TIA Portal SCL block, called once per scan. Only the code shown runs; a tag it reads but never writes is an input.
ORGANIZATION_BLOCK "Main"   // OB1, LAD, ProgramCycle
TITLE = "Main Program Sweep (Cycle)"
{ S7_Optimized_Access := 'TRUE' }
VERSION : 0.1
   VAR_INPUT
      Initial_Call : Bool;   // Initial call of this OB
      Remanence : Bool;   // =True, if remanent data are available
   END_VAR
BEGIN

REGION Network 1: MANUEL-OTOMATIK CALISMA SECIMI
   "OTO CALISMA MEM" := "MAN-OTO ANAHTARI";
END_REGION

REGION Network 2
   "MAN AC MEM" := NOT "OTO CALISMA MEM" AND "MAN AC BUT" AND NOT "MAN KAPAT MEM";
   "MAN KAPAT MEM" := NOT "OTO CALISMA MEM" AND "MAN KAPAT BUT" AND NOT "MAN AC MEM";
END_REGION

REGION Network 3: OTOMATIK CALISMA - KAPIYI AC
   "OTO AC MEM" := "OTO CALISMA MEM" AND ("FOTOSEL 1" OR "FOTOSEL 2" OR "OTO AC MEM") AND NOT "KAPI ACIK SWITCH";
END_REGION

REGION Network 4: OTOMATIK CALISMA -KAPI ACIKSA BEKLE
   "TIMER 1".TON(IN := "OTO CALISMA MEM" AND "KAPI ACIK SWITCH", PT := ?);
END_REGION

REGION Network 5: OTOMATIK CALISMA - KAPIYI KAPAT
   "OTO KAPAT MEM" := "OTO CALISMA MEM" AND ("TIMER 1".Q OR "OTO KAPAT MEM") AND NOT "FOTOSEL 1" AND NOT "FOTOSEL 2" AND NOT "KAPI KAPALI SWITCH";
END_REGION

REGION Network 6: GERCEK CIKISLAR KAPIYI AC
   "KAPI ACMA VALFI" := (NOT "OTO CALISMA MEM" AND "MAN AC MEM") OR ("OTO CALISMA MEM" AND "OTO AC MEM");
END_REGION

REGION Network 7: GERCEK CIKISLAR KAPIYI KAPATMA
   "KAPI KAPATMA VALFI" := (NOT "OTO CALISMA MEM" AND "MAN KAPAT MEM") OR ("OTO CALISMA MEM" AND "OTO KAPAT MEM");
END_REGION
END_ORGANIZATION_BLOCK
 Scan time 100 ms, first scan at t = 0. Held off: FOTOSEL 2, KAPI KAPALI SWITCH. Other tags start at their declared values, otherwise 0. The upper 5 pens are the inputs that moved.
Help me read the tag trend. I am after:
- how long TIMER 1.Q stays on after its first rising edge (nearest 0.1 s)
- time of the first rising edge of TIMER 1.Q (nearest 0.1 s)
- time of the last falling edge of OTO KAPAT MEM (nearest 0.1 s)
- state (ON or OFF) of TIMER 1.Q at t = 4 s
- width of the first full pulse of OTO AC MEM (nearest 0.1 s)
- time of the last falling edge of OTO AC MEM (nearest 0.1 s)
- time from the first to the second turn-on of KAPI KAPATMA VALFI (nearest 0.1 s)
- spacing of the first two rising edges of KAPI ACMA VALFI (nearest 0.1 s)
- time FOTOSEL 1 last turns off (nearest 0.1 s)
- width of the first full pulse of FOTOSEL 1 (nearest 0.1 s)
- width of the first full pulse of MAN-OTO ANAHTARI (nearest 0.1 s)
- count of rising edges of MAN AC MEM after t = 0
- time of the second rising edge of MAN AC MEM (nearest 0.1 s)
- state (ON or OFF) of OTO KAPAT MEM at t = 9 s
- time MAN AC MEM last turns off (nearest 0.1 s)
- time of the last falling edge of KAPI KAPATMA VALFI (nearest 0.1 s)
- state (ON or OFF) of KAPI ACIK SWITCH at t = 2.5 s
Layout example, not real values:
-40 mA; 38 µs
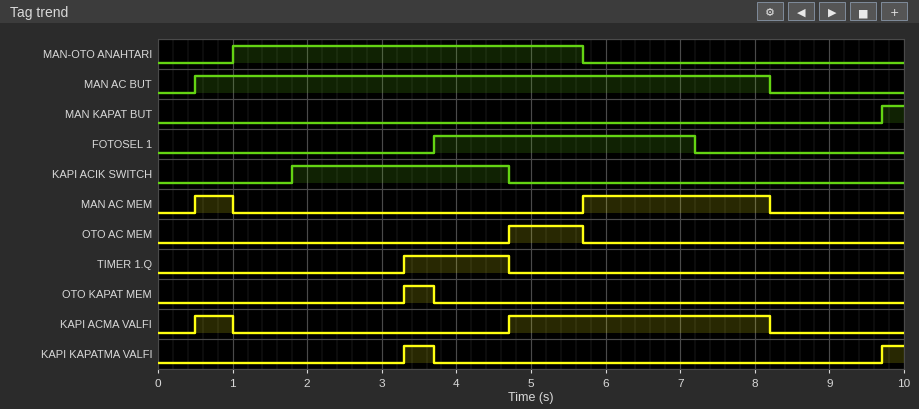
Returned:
1.4 s; 3.3 s; 3.7 s; ON; 1.0 s; 5.7 s; 6.4 s; 4.2 s; 7.2 s; 3.5 s; 4.7 s; 2; 5.7 s; OFF; 8.2 s; 3.7 s; ON
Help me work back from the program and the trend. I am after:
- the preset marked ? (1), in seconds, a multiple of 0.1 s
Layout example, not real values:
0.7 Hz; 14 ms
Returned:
1.5 s
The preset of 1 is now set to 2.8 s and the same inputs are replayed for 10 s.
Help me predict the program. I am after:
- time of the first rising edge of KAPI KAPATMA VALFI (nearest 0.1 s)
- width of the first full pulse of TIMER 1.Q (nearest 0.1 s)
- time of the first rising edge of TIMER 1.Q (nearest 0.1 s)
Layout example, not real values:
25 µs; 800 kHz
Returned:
9.7 s; 0.1 s; 4.6 s
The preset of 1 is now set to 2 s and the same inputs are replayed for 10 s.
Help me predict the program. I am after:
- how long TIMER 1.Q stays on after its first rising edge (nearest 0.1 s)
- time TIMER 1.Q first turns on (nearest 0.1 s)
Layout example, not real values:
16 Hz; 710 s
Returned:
0.9 s; 3.8 s
